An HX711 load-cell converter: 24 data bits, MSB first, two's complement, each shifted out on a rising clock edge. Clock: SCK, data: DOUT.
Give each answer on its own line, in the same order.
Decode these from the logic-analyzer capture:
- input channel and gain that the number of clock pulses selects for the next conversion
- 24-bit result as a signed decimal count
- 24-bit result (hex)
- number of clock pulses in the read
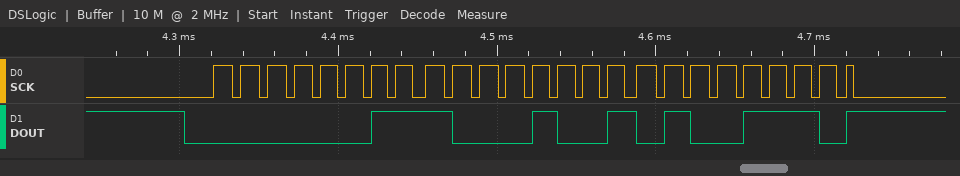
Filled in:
channel A, gain 128
231758
0x03894E
25
